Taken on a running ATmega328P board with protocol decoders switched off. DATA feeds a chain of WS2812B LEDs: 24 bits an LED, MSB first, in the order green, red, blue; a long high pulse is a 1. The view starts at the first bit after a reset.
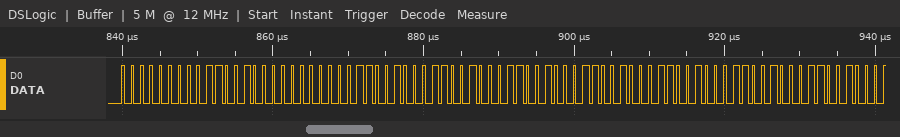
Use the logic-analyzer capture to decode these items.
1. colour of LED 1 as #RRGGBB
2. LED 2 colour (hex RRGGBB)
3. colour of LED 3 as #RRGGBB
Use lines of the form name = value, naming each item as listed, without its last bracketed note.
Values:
colour of LED 1 as #RRGGBB = #640000
LED 2 colour = #646464
colour of LED 3 as #RRGGBB = #646464
